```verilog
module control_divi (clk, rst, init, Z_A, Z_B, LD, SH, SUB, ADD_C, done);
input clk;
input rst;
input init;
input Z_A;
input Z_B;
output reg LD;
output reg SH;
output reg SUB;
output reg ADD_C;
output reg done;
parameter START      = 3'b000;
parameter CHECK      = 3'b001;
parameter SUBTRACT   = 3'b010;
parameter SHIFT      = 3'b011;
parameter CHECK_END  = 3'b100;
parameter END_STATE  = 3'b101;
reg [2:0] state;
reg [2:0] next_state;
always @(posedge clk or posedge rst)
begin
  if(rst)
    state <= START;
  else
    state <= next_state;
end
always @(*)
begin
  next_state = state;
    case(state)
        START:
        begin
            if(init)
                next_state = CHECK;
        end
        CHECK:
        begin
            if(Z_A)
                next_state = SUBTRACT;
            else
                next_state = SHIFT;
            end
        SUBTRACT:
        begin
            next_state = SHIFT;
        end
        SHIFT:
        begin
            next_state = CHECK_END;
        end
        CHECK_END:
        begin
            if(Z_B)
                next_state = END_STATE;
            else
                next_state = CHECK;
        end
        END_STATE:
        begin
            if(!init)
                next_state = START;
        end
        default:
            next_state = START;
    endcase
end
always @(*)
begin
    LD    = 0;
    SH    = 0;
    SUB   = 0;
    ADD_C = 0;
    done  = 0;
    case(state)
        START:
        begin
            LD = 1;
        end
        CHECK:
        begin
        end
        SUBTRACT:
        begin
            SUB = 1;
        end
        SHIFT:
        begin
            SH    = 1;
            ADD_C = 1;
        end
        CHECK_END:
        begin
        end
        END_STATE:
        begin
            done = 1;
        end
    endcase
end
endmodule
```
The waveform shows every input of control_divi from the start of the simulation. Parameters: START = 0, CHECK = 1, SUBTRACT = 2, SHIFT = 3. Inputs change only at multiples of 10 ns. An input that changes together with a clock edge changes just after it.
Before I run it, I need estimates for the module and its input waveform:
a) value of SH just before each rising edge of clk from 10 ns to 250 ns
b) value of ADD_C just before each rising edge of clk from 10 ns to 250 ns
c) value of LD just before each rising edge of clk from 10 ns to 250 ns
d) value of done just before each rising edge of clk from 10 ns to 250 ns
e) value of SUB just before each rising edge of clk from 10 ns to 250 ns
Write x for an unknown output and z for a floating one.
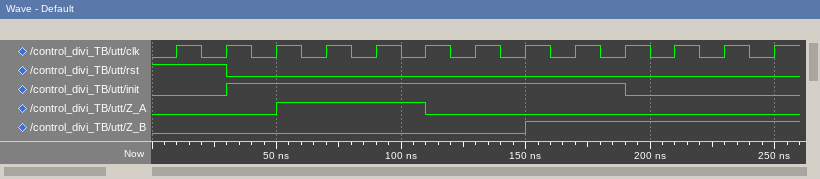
0 0 0 0 0 1 0 0 1 0 0 0 0
0 0 0 0 0 1 0 0 1 0 0 0 0
1 1 1 0 0 0 0 0 0 0 0 1 1
0 0 0 0 0 0 0 0 0 0 1 0 0
0 0 0 0 1 0 0 0 0 0 0 0 0
